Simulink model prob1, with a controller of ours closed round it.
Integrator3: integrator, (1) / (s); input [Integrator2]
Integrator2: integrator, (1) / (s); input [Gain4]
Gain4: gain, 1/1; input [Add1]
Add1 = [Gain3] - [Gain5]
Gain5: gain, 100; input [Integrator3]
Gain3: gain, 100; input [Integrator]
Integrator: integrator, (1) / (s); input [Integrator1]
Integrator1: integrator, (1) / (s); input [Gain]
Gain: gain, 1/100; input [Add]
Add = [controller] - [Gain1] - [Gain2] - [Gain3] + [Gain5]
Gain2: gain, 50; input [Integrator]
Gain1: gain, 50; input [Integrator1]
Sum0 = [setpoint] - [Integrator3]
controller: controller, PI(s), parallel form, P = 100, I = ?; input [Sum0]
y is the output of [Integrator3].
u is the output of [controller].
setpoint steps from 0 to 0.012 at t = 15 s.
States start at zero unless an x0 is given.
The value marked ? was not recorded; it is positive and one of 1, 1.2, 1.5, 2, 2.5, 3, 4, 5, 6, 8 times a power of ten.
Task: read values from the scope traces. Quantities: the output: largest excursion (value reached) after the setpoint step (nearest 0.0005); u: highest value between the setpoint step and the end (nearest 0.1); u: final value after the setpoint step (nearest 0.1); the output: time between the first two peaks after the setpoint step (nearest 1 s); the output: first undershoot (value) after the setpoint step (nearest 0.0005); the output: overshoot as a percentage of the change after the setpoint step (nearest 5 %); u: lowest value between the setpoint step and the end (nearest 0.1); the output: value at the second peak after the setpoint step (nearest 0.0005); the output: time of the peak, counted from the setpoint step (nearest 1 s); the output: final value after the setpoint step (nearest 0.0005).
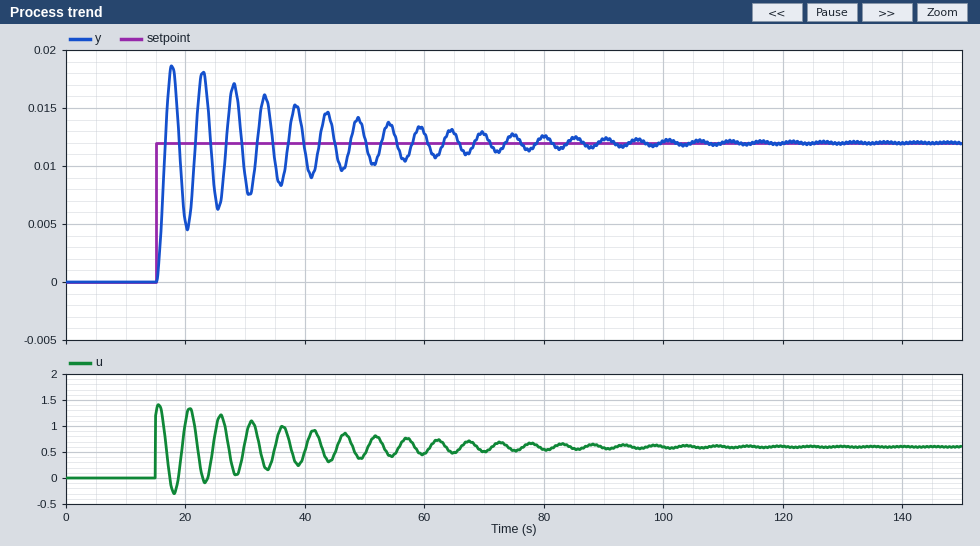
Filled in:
0.0185
1.4
0.6
5 s
0.0045
55 %
-0.3
0.0180
3 s
0.0120
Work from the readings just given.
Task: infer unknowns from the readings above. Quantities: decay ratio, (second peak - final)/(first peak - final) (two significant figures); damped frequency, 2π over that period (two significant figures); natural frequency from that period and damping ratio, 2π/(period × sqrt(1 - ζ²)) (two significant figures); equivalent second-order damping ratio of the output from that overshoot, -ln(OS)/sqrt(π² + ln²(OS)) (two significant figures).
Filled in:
0.92
1.3 rad/s
1.3 rad/s
0.19
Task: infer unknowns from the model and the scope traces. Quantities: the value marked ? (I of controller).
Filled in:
60
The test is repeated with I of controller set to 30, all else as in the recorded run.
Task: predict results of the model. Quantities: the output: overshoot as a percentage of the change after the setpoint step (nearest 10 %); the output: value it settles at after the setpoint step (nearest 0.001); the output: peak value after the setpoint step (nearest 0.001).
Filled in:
30 %
0.012
0.016
